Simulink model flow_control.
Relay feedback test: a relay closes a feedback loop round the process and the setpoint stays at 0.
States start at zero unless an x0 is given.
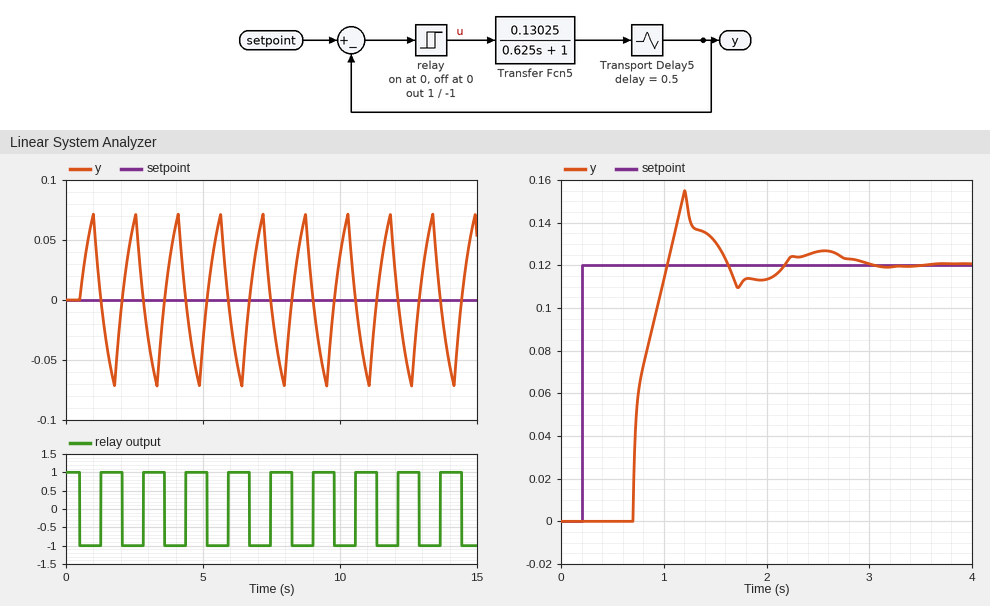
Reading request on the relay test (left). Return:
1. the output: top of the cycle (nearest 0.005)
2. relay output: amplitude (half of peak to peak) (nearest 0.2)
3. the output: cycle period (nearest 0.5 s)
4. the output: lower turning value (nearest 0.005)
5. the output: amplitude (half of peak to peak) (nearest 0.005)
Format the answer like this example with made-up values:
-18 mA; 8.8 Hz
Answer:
0.070; 1.0; 1.5 s; -0.070; 0.070
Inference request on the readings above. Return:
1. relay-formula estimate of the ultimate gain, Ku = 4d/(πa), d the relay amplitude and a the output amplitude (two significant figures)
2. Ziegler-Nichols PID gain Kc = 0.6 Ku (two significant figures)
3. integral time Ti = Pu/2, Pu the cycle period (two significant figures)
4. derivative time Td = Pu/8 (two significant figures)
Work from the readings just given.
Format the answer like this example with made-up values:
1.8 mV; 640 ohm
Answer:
18; 11; 0.75 s; 0.19 s
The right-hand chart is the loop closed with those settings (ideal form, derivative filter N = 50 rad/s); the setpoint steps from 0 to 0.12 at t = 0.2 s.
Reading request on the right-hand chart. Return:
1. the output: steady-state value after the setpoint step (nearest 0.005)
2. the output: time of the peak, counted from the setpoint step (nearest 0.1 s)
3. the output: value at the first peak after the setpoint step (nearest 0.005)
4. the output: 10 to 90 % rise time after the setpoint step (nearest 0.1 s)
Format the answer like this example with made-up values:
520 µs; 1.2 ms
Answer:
0.120; 1.0 s; 0.155; 0.3 s
